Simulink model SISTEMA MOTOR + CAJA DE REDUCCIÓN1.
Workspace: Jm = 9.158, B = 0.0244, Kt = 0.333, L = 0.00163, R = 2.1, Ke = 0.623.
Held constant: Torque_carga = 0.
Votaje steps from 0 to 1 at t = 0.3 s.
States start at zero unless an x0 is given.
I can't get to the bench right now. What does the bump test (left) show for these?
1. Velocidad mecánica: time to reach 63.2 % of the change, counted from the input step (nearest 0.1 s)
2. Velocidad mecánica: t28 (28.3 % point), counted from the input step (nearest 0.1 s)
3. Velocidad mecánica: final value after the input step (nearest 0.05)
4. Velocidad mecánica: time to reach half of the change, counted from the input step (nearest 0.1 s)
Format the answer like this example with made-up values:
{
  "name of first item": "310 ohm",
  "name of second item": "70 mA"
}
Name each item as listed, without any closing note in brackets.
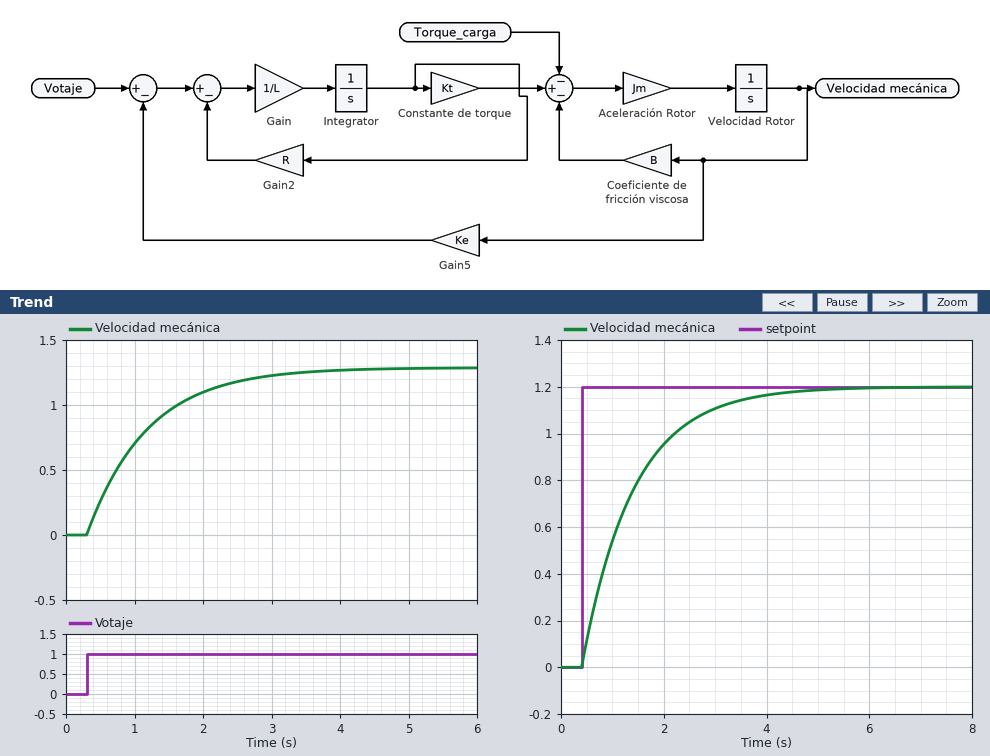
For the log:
{
  "Velocidad mecánica: time to reach 63.2 % of the change, counted from the input step": "0.9 s",
  "Velocidad mecánica: t28 (28.3 % point), counted from the input step": "0.3 s",
  "Velocidad mecánica: final value after the input step": "1.30",
  "Velocidad mecánica: time to reach half of the change, counted from the input step": "0.6 s"
}
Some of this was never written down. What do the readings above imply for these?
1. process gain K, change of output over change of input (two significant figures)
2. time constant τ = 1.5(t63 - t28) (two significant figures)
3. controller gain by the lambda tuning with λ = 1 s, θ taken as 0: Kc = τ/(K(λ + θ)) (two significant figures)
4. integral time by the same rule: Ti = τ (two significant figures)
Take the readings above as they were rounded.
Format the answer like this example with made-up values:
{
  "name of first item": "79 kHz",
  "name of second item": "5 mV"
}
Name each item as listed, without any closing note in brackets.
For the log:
{
  "process gain K, change of output over change of input": "1.3",
  "time constant τ = 1.5(t63 - t28)": "0.90 s",
  "controller gain by the lambda tuning with λ = 1 s, θ taken as 0: Kc = τ/(K(λ + θ))": "0.69",
  "integral time by the same rule: Ti = τ": "0.90 s"
}
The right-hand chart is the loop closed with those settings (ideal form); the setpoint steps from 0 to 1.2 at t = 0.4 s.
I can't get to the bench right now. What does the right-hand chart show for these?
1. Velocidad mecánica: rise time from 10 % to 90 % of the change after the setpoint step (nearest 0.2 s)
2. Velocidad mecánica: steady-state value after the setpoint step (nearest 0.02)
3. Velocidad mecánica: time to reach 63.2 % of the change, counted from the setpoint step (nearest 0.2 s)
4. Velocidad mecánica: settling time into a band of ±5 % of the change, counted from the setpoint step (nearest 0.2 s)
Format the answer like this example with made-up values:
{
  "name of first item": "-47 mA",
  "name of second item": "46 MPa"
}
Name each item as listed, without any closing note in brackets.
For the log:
{
  "Velocidad mecánica: rise time from 10 % to 90 % of the change after the setpoint step": "2.2 s",
  "Velocidad mecánica: steady-state value after the setpoint step": "1.20",
  "Velocidad mecánica: time to reach 63.2 % of the change, counted from the setpoint step": "1.0 s",
  "Velocidad mecánica: settling time into a band of ±5 % of the change, counted from the setpoint step": "3.0 s"
}
